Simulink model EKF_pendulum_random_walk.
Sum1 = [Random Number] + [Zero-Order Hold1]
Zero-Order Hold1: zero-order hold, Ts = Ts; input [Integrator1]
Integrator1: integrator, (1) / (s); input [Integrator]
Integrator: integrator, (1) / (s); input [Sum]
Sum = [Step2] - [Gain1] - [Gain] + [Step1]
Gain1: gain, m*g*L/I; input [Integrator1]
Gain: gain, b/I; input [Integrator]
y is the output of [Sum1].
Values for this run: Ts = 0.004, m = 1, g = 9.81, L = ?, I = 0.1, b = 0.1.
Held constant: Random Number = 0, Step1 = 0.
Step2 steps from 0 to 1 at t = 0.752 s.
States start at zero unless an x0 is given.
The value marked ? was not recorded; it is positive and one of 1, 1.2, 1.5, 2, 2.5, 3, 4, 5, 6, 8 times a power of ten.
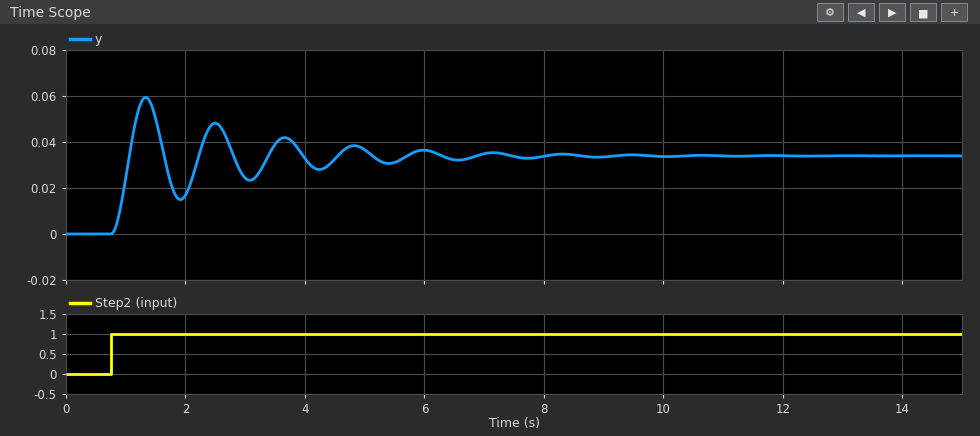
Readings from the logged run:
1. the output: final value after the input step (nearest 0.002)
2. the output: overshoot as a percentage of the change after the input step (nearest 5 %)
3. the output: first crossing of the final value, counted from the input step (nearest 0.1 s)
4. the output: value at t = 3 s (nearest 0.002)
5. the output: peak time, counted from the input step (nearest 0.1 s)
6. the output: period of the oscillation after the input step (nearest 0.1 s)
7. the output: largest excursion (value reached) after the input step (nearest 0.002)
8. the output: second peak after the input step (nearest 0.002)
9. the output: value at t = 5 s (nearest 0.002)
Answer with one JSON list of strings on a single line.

["0.034", "75 %", "0.3 s", "0.024", "0.6 s", "1.2 s", "0.060", "0.048", "0.036"]
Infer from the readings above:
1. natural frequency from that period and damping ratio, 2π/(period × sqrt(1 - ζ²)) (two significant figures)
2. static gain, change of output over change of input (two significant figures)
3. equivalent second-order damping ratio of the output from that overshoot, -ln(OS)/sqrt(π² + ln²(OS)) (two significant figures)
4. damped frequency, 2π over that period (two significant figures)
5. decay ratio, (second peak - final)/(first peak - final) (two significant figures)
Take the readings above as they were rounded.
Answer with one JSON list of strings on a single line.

["5.3 rad/s", "0.034", "0.091", "5.2 rad/s", "0.54"]
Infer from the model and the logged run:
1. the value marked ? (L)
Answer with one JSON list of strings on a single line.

["0.3"]
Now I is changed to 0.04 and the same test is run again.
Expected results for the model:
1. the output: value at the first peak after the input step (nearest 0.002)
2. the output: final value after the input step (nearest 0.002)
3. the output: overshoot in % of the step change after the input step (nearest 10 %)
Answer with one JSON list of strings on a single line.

["0.022", "0.014", "60 %"]
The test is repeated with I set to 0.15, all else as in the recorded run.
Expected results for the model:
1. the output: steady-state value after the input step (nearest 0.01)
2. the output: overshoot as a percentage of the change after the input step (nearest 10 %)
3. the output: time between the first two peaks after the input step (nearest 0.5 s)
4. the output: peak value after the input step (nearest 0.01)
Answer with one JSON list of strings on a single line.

["0.05", "80 %", "1.5 s", "0.09"]
